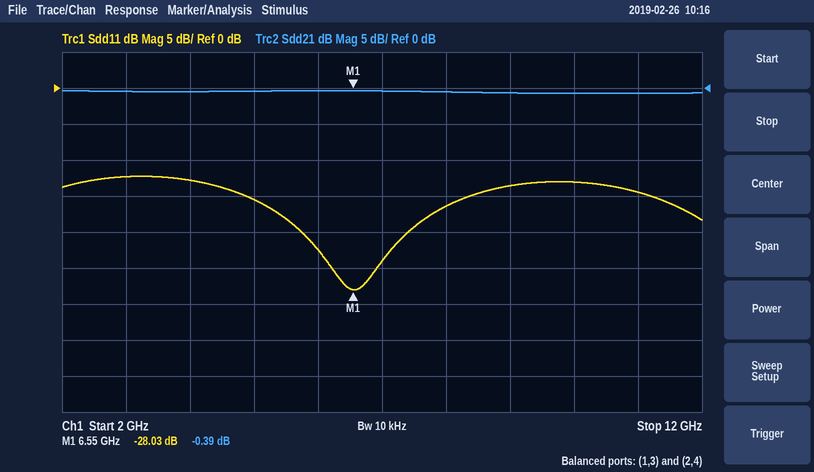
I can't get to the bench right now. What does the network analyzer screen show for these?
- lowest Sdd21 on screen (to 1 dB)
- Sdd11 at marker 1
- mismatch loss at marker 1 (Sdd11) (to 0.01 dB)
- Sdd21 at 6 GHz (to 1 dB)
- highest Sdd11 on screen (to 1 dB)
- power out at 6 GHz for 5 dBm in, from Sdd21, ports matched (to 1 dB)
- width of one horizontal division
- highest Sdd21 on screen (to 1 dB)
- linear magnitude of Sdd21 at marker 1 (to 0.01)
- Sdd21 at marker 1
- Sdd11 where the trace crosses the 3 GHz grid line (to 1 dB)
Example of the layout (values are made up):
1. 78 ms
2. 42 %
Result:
1. -1 dB
2. -28.03 dB
3. 0.01 dB
4. 0 dB
5. -12 dB
6. 5 dBm
7. 1 GHz
8. 0 dB
9. 0.96
10. -0.39 dB
11. -12 dB
